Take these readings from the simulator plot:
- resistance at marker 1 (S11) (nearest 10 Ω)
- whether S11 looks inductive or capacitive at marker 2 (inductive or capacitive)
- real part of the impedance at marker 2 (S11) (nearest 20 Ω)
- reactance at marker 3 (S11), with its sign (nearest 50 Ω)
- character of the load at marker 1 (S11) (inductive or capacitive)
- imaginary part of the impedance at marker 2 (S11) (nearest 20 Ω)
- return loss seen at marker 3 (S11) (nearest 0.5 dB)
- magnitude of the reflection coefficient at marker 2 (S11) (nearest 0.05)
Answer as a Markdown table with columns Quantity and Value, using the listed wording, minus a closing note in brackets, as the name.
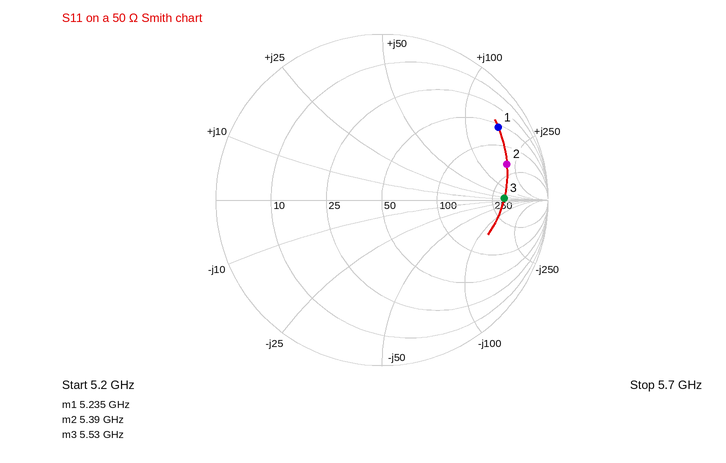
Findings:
| Quantity | Value |
|---|---|
| resistance at marker 1 (S11) | 60 Ω |
| whether S11 looks inductive or capacitive at marker 2 | inductive |
| real part of the impedance at marker 2 (S11) | 180 Ω |
| reactance at marker 3 (S11), with its sign | 0 Ω |
| character of the load at marker 1 (S11) | inductive |
| imaginary part of the impedance at marker 2 (S11) | +200 Ω |
| return loss seen at marker 3 (S11) | 2.5 dB |
| magnitude of the reflection coefficient at marker 2 (S11) | 0.80 |
